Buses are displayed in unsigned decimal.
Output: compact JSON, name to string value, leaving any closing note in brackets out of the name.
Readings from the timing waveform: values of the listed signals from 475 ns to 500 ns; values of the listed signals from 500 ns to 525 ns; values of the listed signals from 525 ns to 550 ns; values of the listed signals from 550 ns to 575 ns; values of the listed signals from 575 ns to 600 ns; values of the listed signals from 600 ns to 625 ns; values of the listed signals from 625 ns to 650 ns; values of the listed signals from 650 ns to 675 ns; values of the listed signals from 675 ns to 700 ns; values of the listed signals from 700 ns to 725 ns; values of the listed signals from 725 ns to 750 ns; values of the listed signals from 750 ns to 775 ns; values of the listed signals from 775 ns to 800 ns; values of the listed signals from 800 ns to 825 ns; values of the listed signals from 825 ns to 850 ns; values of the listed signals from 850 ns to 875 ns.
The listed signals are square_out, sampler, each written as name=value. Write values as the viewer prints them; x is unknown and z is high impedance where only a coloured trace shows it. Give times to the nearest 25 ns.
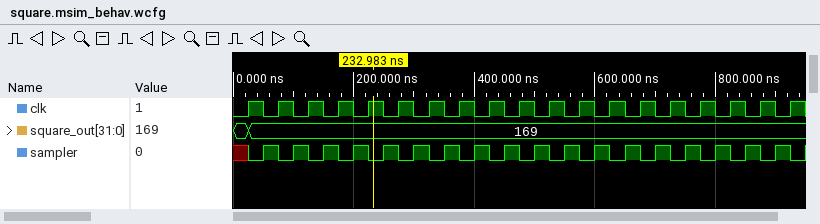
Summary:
{"values of the listed signals from 475 ns to 500 ns": "square_out=169, sampler=0", "values of the listed signals from 500 ns to 525 ns": "square_out=169, sampler=1", "values of the listed signals from 525 ns to 550 ns": "square_out=169, sampler=0", "values of the listed signals from 550 ns to 575 ns": "square_out=169, sampler=1", "values of the listed signals from 575 ns to 600 ns": "square_out=169, sampler=0", "values of the listed signals from 600 ns to 625 ns": "square_out=169, sampler=1", "values of the listed signals from 625 ns to 650 ns": "square_out=169, sampler=0", "values of the listed signals from 650 ns to 675 ns": "square_out=169, sampler=1", "values of the listed signals from 675 ns to 700 ns": "square_out=169, sampler=0", "values of the listed signals from 700 ns to 725 ns": "square_out=169, sampler=1", "values of the listed signals from 725 ns to 750 ns": "square_out=169, sampler=0", "values of the listed signals from 750 ns to 775 ns": "square_out=169, sampler=1", "values of the listed signals from 775 ns to 800 ns": "square_out=169, sampler=0", "values of the listed signals from 800 ns to 825 ns": "square_out=169, sampler=1", "values of the listed signals from 825 ns to 850 ns": "square_out=169, sampler=0", "values of the listed signals from 850 ns to 875 ns": "square_out=169, sampler=1"}
